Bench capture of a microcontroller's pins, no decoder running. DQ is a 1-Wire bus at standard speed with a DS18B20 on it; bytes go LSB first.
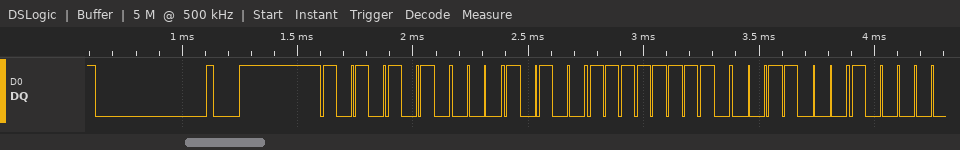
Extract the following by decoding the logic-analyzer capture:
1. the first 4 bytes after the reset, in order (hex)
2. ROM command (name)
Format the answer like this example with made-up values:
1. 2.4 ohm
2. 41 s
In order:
1. 55 28 FF 18
2. Match ROM
